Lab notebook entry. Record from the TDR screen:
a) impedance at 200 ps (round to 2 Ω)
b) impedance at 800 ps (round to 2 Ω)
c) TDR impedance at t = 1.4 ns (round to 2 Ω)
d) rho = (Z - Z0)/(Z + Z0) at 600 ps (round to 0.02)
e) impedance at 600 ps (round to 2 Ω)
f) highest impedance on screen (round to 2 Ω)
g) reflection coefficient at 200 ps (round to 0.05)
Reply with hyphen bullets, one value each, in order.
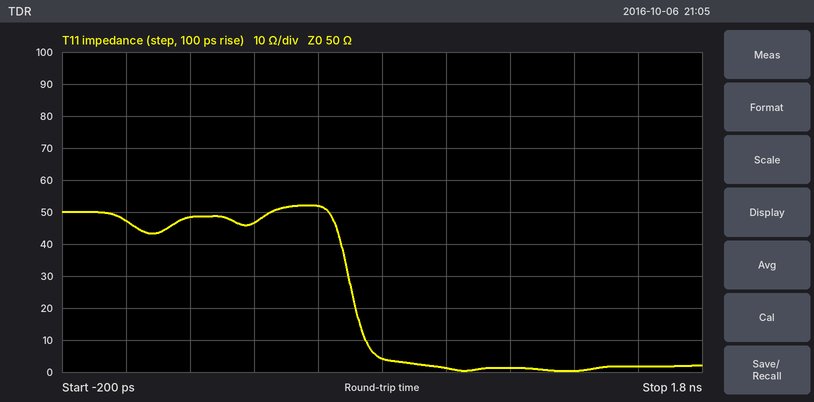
- 48 Ω
- 4 Ω
- 0 Ω
- +0.02
- 52 Ω
- 52 Ω
- 0.00
